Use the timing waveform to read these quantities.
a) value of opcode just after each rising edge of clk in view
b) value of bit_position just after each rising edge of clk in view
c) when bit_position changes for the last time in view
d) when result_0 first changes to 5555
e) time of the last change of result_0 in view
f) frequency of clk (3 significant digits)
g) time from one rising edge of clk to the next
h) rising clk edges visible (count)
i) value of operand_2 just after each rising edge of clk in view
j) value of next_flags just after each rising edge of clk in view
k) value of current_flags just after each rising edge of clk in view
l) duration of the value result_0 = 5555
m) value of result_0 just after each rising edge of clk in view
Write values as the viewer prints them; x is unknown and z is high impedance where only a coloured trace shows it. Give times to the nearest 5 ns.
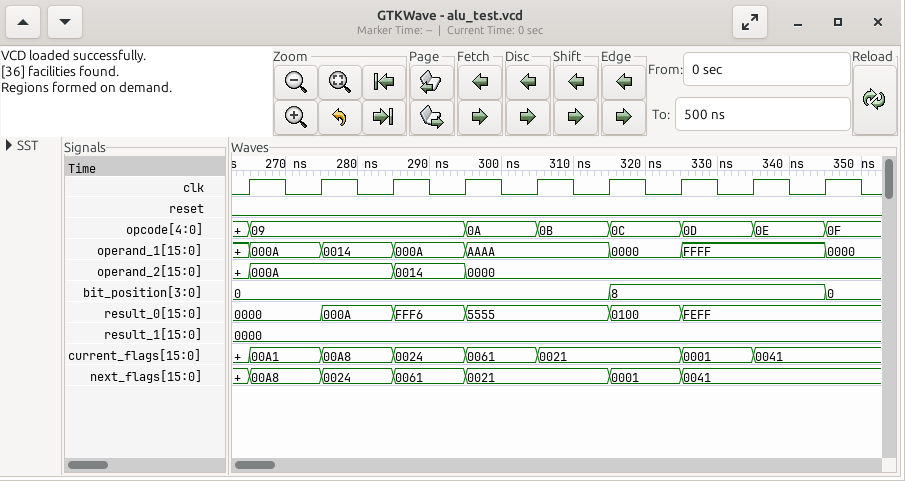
09, 09, 09, 0A, 0B, 0C, 0D, 0E, 0F
0, 0, 0, 0, 0, 8, 8, 8, 0
345 ns
295 ns
325 ns
100 MHz
10 ns
9
000A, 000A, 0014, 0000, 0000, 0000, 0000, 0000, 0000
00A8, 0024, 0061, 0021, 0021, 0001, 0041, 0041, 0041
00A1, 00A8, 0024, 0061, 0021, 0021, 0001, 0041, 0041
20 ns
0000, 000A, FFF6, 5555, 5555, 0100, FEFF, FEFF, FEFF
